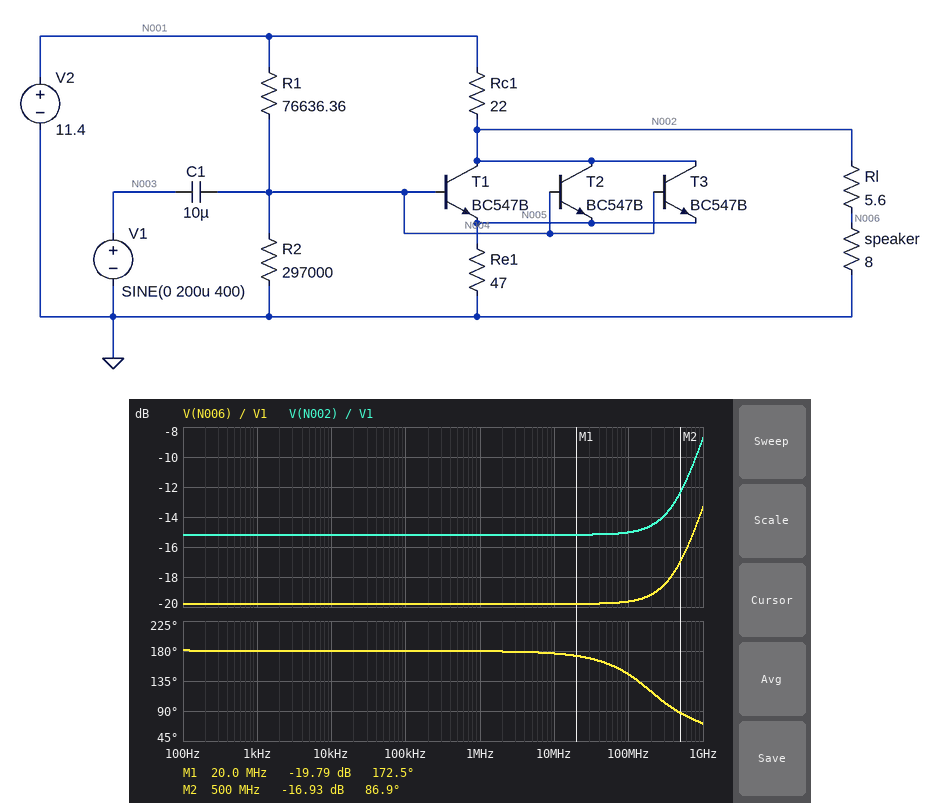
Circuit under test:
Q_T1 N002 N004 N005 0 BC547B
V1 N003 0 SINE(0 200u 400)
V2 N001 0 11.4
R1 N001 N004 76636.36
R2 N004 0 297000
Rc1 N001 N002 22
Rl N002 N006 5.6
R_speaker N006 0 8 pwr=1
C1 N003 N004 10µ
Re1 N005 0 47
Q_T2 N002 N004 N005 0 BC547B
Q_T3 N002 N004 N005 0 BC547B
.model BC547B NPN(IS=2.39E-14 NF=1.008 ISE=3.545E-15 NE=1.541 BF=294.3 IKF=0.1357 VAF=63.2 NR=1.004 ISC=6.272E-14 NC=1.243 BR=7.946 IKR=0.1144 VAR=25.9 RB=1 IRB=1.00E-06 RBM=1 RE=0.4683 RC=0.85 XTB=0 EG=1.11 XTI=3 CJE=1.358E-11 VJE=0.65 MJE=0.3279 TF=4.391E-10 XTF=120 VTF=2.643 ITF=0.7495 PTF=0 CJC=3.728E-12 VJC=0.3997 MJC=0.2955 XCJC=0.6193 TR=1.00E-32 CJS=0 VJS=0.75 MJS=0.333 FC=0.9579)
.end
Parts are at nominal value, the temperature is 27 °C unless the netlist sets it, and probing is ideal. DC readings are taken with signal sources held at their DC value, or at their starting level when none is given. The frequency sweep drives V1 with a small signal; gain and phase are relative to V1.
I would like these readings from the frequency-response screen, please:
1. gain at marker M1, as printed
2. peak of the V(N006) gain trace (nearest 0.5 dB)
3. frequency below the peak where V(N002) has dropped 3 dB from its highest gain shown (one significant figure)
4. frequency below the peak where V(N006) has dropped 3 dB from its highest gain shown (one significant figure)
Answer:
-19.79 dB
-13.5 dB
600 MHz
600 MHz
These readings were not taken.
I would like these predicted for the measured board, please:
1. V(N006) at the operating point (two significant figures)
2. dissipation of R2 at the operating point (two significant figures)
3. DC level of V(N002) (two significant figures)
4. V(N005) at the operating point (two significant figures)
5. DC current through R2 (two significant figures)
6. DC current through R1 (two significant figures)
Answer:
2.4 V
16 µW
4.1 V
1.5 V
7.3 µA
120 µA
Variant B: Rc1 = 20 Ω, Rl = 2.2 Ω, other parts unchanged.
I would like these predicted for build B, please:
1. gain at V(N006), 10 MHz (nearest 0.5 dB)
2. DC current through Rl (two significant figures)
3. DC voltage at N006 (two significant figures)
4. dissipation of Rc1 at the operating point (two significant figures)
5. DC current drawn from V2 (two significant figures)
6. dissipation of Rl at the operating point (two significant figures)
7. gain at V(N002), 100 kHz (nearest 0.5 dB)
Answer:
-19.0 dB
360 mA
2.9 V
3.0 W
390 mA
280 mW
-17.0 dB
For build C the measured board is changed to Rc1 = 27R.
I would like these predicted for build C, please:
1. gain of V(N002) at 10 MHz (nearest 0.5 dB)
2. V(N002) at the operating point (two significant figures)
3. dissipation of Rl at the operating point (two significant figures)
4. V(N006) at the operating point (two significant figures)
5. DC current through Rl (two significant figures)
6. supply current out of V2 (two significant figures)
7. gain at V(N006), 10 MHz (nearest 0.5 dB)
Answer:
-14.5 dB
3.5 V
380 mW
2.1 V
260 mA
290 mA
-19.0 dB
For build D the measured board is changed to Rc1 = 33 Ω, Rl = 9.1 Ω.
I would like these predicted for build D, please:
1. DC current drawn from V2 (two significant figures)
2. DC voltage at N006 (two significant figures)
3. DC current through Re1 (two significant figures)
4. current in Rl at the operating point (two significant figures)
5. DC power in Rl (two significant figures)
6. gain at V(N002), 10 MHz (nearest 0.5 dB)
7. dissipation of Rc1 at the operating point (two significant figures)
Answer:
240 mA
1.7 V
31 mA
210 mA
390 mW
-12.5 dB
1.9 W
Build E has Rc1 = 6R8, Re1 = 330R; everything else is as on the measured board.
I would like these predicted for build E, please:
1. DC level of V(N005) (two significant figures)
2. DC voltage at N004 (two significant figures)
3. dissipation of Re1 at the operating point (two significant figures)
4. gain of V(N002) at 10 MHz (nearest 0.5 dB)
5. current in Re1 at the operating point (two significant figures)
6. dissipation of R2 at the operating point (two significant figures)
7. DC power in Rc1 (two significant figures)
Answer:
5.1 V
5.8 V
78 mW
-37.0 dB
15 mA
110 µW
2.2 W
